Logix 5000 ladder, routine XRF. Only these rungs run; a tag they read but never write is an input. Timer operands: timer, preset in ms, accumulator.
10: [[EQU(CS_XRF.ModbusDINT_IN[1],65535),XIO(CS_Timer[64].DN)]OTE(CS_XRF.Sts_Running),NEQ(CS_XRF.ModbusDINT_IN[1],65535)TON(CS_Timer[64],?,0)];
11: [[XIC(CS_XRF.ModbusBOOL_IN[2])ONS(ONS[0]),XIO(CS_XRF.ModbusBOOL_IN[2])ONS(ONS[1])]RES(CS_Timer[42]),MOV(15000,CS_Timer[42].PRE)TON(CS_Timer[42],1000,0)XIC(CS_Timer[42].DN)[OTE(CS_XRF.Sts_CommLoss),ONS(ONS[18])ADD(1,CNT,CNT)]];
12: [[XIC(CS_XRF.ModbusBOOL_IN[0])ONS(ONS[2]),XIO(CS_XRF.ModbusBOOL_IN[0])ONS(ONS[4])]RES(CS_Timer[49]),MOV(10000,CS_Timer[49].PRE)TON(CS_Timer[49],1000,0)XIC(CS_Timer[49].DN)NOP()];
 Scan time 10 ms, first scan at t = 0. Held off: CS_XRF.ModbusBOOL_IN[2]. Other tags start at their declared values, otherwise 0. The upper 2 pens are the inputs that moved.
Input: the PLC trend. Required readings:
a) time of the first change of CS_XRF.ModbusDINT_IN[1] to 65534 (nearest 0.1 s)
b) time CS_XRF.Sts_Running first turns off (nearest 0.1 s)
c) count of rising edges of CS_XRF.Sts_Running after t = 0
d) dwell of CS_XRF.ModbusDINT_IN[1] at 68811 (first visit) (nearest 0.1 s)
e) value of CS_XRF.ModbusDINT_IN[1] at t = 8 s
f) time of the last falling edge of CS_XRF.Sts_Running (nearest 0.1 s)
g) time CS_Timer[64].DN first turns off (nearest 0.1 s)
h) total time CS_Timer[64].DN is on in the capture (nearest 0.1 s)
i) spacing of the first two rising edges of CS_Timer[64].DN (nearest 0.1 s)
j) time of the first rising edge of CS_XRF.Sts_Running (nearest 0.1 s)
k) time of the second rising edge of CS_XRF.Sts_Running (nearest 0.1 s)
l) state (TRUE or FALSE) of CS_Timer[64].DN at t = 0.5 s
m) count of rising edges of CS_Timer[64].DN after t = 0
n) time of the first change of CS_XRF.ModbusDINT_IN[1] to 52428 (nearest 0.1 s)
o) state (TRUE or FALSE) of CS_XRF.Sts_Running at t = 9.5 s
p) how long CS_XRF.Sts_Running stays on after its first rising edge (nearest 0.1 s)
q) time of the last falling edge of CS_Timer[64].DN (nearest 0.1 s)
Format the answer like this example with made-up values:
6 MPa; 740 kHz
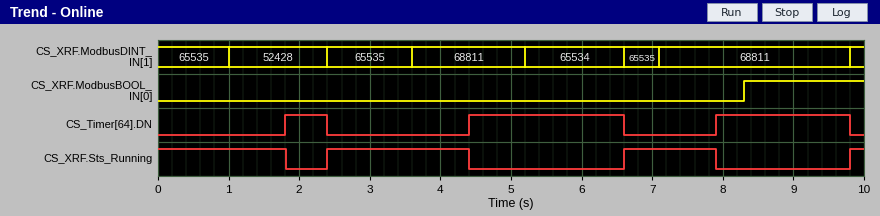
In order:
5.2 s; 1.8 s; 3; 1.6 s; 68811; 7.9 s; 2.4 s; 4.7 s; 2.6 s; 2.4 s; 6.6 s; FALSE; 3; 1.0 s; FALSE; 2.0 s; 9.8 s
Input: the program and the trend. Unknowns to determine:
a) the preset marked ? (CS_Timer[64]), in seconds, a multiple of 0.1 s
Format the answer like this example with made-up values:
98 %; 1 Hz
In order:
0.8 s
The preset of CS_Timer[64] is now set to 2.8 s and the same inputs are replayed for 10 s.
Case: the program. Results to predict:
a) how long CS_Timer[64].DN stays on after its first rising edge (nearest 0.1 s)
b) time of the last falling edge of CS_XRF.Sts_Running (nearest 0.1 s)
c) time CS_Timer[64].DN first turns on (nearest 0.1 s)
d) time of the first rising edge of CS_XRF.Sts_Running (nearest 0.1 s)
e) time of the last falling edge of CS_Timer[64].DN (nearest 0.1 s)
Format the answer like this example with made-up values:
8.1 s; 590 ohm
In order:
0.2 s; 6.4 s; 6.4 s; 6.6 s; 6.6 s
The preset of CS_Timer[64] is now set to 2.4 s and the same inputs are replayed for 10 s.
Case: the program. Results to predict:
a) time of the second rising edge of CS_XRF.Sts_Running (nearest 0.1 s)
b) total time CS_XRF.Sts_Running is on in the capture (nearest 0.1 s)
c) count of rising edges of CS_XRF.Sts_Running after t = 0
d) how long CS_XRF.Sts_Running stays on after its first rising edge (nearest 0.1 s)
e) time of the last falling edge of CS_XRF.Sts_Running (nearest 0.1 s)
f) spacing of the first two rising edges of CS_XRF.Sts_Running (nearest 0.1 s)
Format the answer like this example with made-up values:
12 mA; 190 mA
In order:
9.8 s; 9.1 s; 2; 2.9 s; 9.5 s; 3.2 s
